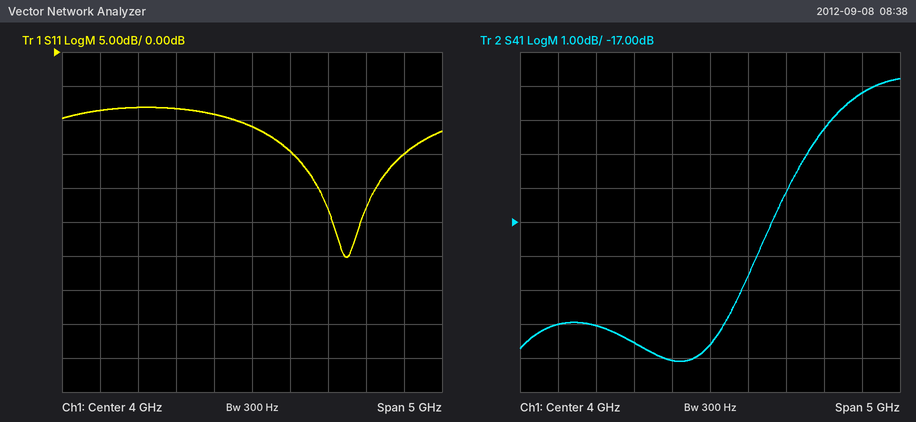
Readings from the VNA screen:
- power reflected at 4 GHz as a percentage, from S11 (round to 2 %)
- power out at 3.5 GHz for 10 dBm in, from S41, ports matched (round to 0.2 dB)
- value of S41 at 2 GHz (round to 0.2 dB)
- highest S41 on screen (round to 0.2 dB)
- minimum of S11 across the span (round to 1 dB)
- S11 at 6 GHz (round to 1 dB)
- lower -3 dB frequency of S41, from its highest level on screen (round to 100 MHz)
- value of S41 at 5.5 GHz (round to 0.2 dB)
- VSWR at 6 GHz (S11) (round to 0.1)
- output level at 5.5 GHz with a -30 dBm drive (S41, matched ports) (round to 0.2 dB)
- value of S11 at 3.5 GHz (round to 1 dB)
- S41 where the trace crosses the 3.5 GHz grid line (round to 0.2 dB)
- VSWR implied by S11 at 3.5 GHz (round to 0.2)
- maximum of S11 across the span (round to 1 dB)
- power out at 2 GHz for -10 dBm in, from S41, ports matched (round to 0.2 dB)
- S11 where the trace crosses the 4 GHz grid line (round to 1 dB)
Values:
8 %
-11.0 dBm
-20.0 dB
-12.8 dB
-30 dB
-15 dB
5.1 GHz
-14.2 dB
1.4
-44.2 dBm
-9 dB
-21.0 dB
2.0
-8 dB
-30.0 dBm
-11 dB
